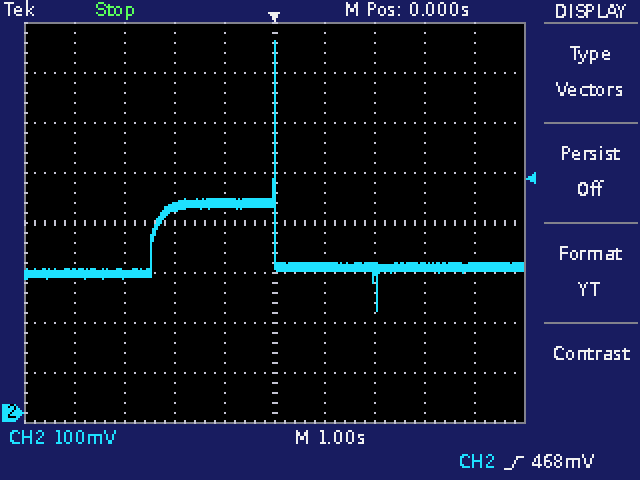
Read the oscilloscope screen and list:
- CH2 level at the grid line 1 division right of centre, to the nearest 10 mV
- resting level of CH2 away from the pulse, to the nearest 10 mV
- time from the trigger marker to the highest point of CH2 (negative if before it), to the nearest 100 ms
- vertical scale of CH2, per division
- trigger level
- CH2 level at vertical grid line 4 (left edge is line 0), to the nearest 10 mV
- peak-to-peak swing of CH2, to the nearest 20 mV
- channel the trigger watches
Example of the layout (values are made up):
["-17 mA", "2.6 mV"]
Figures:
["290 mV", "290 mV", "0.0 s", "100 mV", "468 mV", "420 mV", "540 mV", "CH2"]
